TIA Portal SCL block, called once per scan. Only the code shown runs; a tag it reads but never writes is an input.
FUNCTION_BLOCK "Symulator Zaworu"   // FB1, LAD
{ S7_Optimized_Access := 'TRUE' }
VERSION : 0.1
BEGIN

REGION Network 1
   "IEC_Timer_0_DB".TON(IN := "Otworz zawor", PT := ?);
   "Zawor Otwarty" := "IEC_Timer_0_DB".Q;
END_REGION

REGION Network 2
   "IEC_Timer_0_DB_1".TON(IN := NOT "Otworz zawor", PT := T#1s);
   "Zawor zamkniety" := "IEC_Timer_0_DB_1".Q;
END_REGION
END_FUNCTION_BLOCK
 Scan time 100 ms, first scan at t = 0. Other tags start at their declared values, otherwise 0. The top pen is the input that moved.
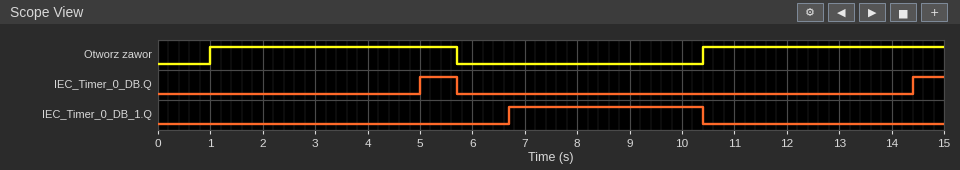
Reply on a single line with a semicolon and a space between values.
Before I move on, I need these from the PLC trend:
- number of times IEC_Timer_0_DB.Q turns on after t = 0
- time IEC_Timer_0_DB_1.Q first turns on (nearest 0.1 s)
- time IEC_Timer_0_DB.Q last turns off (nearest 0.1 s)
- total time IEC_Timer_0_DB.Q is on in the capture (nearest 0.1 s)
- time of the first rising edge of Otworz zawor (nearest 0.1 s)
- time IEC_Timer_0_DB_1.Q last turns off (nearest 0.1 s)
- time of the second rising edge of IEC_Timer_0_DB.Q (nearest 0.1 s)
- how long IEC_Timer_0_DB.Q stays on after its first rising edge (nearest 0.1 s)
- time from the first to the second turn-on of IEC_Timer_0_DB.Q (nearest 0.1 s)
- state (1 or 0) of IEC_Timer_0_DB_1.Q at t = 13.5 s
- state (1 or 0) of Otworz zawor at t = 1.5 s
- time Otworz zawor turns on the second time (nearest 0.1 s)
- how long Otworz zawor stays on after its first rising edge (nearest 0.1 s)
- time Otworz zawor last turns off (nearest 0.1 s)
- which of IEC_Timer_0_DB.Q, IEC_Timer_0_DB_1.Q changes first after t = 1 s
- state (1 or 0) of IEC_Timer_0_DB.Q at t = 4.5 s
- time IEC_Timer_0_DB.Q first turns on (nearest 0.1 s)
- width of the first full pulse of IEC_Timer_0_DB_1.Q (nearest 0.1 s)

2; 6.7 s; 5.7 s; 1.3 s; 1.0 s; 10.4 s; 14.4 s; 0.7 s; 9.4 s; 0; 1; 10.4 s; 4.7 s; 5.7 s; IEC_Timer_0_DB.Q; 0; 5.0 s; 3.7 s
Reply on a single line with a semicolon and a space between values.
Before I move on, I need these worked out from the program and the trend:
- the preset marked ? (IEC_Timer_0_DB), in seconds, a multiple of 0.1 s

4.0 s
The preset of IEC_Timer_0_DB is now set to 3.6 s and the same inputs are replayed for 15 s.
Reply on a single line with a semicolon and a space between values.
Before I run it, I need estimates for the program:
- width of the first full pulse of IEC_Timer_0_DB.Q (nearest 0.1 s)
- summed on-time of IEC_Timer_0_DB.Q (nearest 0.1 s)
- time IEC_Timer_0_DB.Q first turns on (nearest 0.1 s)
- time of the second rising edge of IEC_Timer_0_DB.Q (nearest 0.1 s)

1.1 s; 2.1 s; 4.6 s; 14.0 s
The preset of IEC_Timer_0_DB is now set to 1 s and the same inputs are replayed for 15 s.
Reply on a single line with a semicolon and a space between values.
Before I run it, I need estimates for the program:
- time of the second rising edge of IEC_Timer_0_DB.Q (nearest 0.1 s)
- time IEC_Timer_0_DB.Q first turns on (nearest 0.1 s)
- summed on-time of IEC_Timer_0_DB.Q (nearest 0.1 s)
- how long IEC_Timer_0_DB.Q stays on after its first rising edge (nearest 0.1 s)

11.4 s; 2.0 s; 7.3 s; 3.7 s
